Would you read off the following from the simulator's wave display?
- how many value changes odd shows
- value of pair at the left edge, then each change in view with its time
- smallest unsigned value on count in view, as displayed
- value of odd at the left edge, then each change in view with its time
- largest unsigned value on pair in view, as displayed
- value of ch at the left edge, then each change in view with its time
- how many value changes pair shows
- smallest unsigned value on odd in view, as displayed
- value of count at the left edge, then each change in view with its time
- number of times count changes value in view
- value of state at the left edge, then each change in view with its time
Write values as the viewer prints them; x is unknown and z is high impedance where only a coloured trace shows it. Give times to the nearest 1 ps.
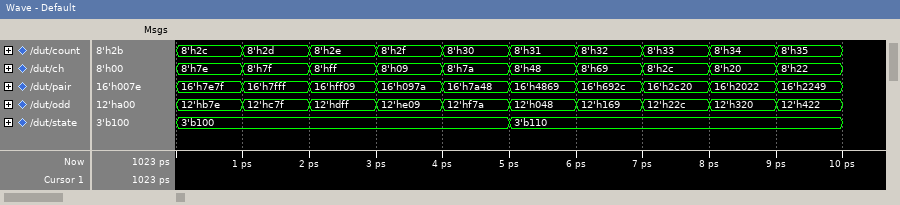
9
16'h7e7f, 16'h7fff at 1 ps, 16'hff09 at 2 ps, 16'h097a at 3 ps, 16'h7a48 at 4 ps, 16'h4869 at 5 ps, 16'h692c at 6 ps, 16'h2c20 at 7 ps, 16'h2022 at 8 ps, 16'h2249 at 9 ps
8'h2c
12'hb7e, 12'hc7f at 1 ps, 12'hdff at 2 ps, 12'he09 at 3 ps, 12'hf7a at 4 ps, 12'h048 at 5 ps, 12'h169 at 6 ps, 12'h22c at 7 ps, 12'h320 at 8 ps, 12'h422 at 9 ps
16'hff09
8'h7e, 8'h7f at 1 ps, 8'hff at 2 ps, 8'h09 at 3 ps, 8'h7a at 4 ps, 8'h48 at 5 ps, 8'h69 at 6 ps, 8'h2c at 7 ps, 8'h20 at 8 ps, 8'h22 at 9 ps
9
12'h048
8'h2c, 8'h2d at 1 ps, 8'h2e at 2 ps, 8'h2f at 3 ps, 8'h30 at 4 ps, 8'h31 at 5 ps, 8'h32 at 6 ps, 8'h33 at 7 ps, 8'h34 at 8 ps, 8'h35 at 9 ps
9
3'b100, 3'b110 at 5 ps
